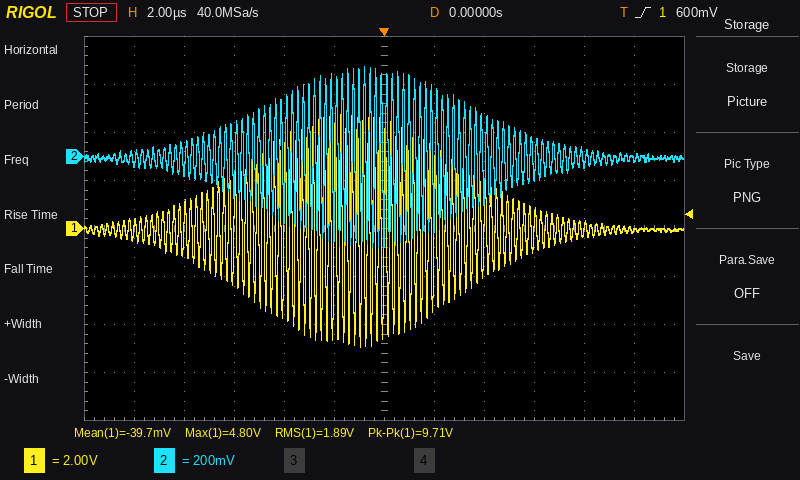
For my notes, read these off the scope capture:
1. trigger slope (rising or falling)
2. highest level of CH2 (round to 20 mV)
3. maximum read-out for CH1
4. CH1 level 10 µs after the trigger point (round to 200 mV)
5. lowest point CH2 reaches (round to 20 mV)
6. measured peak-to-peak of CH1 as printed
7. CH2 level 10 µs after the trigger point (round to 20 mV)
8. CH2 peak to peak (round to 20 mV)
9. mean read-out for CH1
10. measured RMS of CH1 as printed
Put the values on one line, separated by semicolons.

rising; 380 mV; 4.80 V; 0.0 V; -380 mV; 9.71 V; 0 mV; 760 mV; -39.7 mV; 1.89 V
